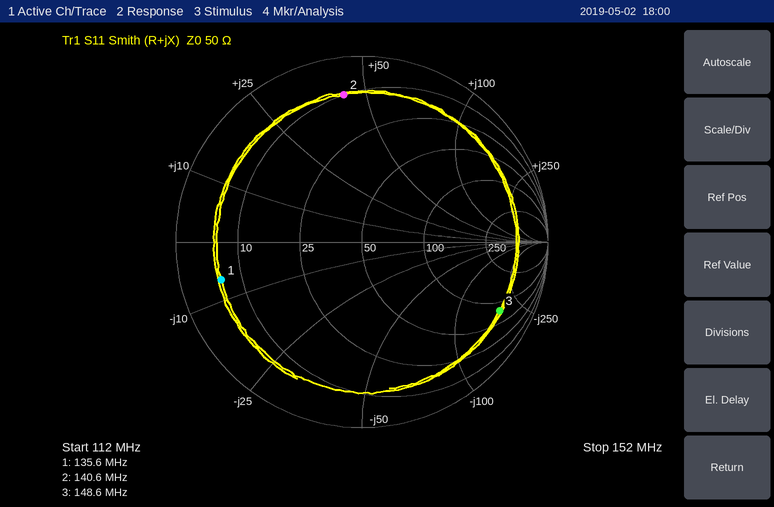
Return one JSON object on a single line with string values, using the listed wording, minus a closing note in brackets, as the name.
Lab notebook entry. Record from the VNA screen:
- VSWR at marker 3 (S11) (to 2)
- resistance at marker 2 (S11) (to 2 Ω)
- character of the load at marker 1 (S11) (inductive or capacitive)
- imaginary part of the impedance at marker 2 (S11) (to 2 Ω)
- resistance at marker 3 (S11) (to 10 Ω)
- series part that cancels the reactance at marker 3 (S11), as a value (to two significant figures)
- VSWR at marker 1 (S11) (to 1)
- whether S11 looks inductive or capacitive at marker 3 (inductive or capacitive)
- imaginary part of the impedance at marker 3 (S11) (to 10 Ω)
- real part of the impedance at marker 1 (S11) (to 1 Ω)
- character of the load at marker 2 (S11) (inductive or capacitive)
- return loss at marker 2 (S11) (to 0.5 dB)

{"VSWR at marker 3 (S11)": "10", "resistance at marker 2 (S11)": "10 Ω", "character of the load at marker 1 (S11)": "capacitive", "imaginary part of the impedance at marker 2 (S11)": "+44 Ω", "resistance at marker 3 (S11)": "80 Ω", "series part that cancels the reactance at marker 3 (S11), as a value": "190 nH", "VSWR at marker 1 (S11)": "8", "whether S11 looks inductive or capacitive at marker 3": "capacitive", "imaginary part of the impedance at marker 3 (S11)": "-180 Ω", "real part of the impedance at marker 1 (S11)": "6 Ω", "character of the load at marker 2 (S11)": "inductive", "return loss at marker 2 (S11)": "2.0 dB"}
